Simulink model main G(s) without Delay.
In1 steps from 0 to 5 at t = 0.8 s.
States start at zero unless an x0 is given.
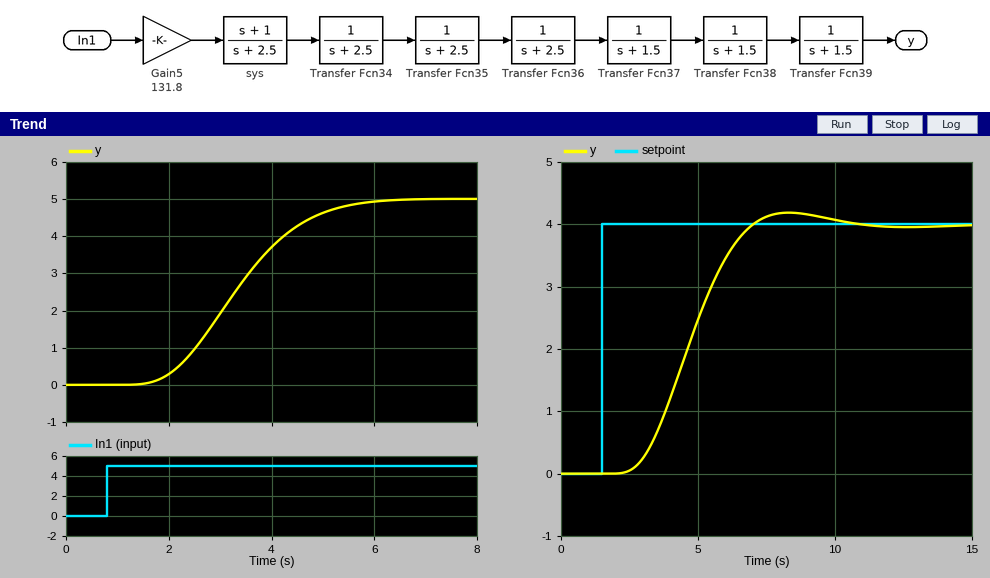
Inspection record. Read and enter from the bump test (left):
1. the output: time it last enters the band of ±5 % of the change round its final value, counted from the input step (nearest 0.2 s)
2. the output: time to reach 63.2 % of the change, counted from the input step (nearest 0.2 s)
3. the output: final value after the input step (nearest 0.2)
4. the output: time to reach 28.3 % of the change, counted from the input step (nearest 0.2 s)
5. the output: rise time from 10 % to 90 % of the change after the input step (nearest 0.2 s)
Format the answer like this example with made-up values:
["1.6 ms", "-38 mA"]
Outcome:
["4.4 s", "2.8 s", "5.0", "2.0 s", "2.6 s"]
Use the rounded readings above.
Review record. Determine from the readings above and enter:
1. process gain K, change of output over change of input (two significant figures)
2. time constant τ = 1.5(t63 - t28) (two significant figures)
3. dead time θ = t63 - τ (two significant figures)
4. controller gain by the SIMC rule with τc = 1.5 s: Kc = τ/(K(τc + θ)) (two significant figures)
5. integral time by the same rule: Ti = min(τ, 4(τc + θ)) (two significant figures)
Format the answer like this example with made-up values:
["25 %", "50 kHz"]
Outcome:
["1.0", "1.2 s", "1.6 s", "0.39", "1.2 s"]
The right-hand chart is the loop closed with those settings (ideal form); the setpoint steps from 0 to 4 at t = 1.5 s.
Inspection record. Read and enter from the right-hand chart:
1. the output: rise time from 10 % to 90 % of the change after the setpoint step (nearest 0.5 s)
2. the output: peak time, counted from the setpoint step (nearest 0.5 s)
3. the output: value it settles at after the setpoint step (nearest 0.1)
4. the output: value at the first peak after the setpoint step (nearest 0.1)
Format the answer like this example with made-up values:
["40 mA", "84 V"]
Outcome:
["3.0 s", "7.0 s", "4.0", "4.2"]
